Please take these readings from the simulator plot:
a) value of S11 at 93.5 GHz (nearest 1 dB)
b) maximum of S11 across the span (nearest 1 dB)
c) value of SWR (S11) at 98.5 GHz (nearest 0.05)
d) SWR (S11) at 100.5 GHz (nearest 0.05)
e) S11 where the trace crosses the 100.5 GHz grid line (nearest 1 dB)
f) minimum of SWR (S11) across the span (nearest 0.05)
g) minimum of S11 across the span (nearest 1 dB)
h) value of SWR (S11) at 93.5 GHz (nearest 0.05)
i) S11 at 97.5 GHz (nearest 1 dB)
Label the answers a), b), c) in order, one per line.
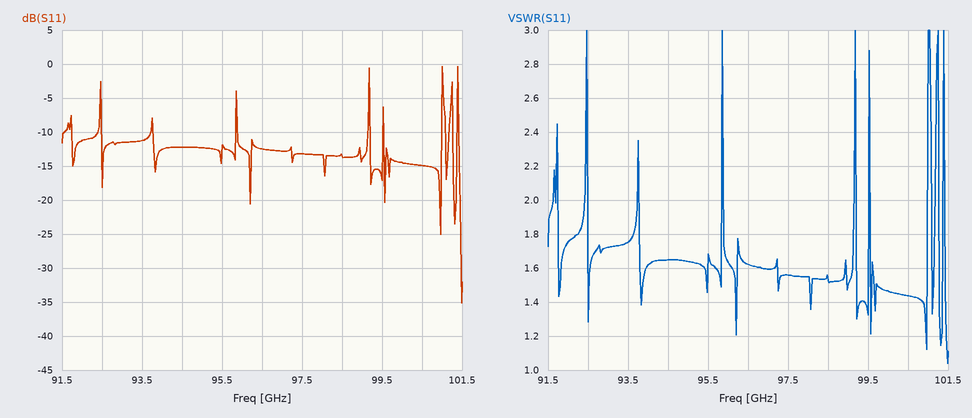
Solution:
a) -11 dB
b) 0 dB
c) 1.55
d) 1.45
e) -15 dB
f) 1.05
g) -35 dB
h) 1.75
i) -13 dB
